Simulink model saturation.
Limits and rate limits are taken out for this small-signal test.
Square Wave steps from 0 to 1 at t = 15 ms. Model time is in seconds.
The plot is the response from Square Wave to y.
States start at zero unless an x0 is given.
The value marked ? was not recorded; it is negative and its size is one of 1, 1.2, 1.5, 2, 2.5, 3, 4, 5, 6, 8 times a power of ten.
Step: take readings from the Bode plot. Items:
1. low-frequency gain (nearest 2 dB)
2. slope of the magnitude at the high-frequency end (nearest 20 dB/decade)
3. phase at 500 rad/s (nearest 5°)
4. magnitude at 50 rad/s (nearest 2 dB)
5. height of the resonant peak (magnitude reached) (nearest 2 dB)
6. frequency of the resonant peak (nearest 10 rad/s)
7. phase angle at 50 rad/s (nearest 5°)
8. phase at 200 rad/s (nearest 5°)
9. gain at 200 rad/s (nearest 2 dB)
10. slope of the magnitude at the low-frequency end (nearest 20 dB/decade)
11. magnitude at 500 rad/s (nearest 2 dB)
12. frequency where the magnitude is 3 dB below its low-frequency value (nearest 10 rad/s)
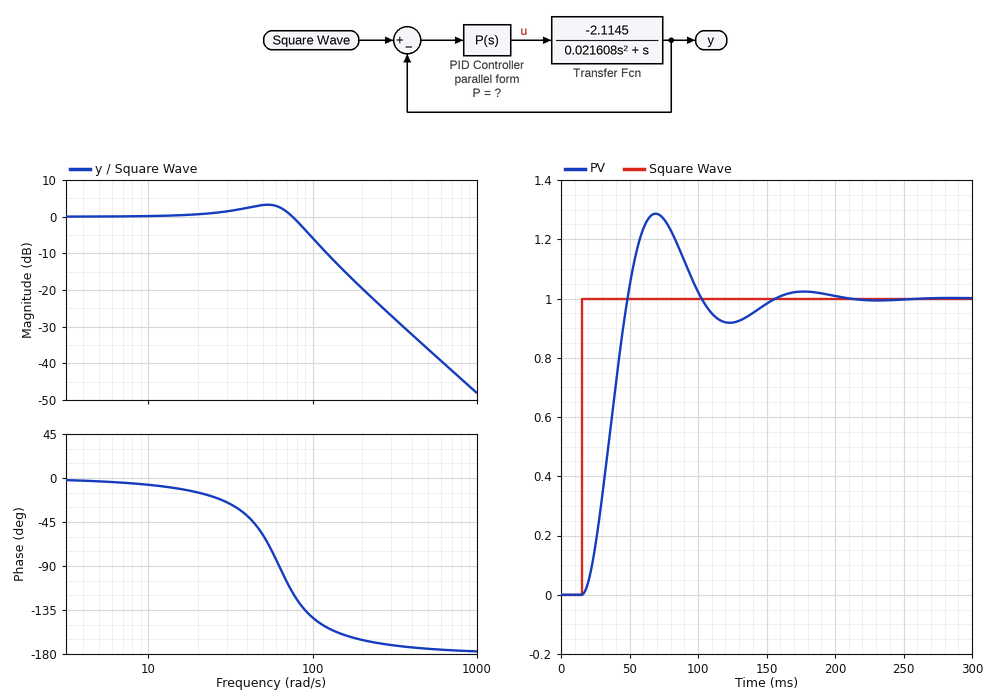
0 dB
-40 dB/decade
-175°
4 dB
4 dB
50 rad/s
-60°
-165°
-20 dB
0 dB/decade
-36 dB
90 rad/s
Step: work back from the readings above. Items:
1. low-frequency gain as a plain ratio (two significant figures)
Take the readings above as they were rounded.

1.0
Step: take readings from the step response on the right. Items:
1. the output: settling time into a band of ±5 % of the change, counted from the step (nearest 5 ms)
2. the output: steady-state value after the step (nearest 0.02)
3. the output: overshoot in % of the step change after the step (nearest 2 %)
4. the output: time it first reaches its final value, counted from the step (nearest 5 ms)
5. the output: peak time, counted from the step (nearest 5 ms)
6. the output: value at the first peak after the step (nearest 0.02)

125 ms
1.00
28 %
35 ms
55 ms
1.28
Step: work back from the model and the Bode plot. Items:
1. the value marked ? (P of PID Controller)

-40
